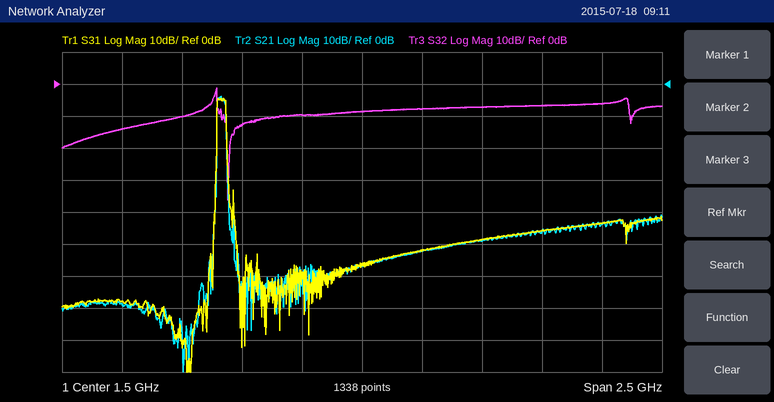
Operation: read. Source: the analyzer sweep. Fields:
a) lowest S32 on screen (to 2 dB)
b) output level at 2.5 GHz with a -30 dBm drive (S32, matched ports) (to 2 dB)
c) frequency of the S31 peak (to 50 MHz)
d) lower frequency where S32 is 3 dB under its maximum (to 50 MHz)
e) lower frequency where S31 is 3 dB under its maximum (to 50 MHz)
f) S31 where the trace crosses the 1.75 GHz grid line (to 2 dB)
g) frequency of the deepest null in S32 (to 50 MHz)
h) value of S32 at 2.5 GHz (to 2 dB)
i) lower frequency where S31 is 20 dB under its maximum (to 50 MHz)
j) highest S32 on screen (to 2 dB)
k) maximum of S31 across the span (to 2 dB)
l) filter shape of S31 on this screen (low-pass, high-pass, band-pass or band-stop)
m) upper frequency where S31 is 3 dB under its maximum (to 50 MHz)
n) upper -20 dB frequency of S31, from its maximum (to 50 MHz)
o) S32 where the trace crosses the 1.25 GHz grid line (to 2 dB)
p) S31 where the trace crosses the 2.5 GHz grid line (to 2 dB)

-36 dB
-36 dBm
900 MHz
900 MHz
900 MHz
-52 dB
950 MHz
-6 dB
900 MHz
-2 dB
-4 dB
band-pass
950 MHz
950 MHz
-10 dB
-44 dB
